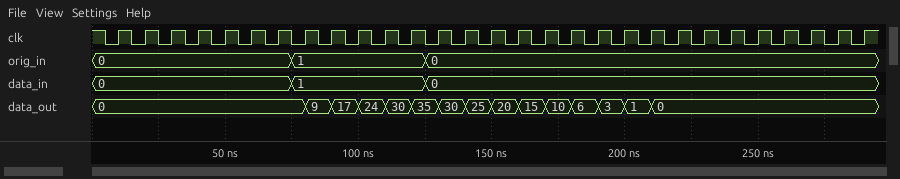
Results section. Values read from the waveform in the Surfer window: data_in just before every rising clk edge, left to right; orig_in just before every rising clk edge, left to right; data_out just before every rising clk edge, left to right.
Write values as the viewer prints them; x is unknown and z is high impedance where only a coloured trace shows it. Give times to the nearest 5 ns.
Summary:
0, 0, 0, 0, 0, 0, 0, 1, 1, 1, 1, 1, 0, 0, 0, 0, 0, 0, 0, 0, 0, 0, 0, 0, 0, 0, 0, 0, 0
0, 0, 0, 0, 0, 0, 0, 1, 1, 1, 1, 1, 0, 0, 0, 0, 0, 0, 0, 0, 0, 0, 0, 0, 0, 0, 0, 0, 0
0, 0, 0, 0, 0, 0, 0, 0, 9, 17, 24, 30, 35, 30, 25, 20, 15, 10, 6, 3, 1, 0, 0, 0, 0, 0, 0, 0, 0
